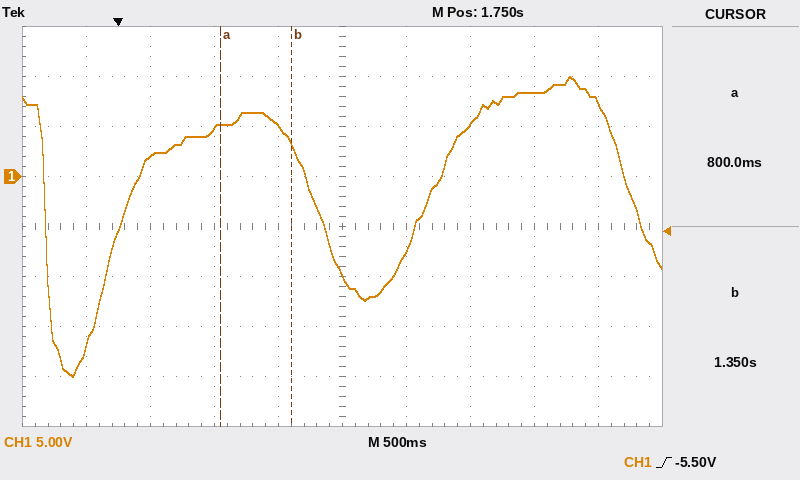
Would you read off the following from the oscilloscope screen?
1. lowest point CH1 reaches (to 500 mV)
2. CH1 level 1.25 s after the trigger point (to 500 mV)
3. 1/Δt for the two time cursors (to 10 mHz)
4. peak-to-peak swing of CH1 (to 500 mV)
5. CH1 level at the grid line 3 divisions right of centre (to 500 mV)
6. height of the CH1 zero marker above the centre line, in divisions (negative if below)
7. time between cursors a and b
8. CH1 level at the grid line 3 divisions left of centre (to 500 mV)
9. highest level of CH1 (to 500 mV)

-20.0 V
5.0 V
1.82 Hz
30.0 V
8.5 V
+1.0 div
550 ms
2.0 V
10.0 V
